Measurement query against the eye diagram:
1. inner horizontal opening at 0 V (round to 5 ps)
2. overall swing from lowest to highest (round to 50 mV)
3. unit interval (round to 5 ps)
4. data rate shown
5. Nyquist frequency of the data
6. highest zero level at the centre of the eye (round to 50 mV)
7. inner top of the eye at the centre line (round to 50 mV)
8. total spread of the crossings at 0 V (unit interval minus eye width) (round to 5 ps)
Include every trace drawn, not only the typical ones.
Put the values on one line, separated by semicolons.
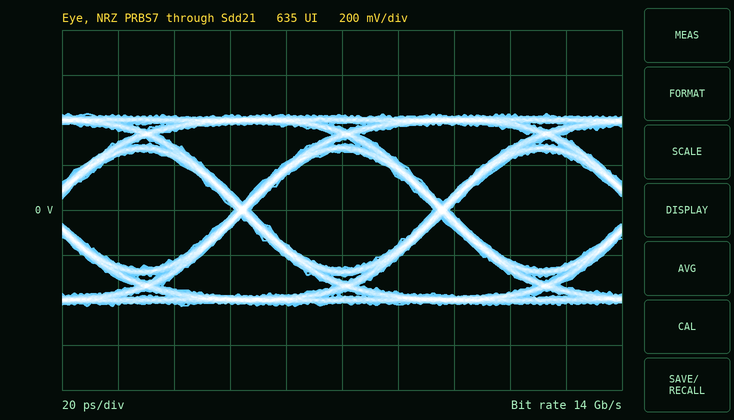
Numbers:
65 ps; 850 mV; 70 ps; 14 Gb/s; 7 GHz; -250 mV; 250 mV; 5 ps
